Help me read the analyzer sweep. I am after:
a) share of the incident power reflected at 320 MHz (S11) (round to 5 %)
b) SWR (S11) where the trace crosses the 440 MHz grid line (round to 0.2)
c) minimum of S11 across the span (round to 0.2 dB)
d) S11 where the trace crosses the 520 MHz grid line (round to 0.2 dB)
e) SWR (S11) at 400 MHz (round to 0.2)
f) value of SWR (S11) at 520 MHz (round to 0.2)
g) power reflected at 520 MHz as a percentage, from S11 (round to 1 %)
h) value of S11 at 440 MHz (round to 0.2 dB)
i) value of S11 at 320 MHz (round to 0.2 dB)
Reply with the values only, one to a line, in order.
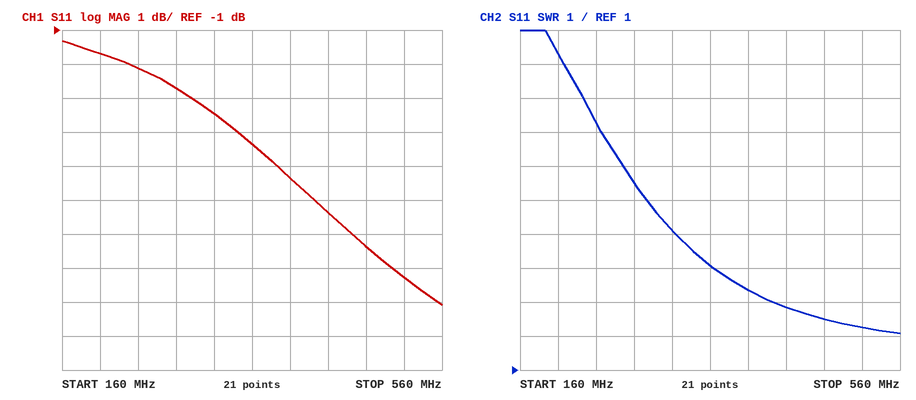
45 %
2.8
-9.0 dB
-8.2 dB
3.4
2.2
15 %
-6.4 dB
-3.4 dB
